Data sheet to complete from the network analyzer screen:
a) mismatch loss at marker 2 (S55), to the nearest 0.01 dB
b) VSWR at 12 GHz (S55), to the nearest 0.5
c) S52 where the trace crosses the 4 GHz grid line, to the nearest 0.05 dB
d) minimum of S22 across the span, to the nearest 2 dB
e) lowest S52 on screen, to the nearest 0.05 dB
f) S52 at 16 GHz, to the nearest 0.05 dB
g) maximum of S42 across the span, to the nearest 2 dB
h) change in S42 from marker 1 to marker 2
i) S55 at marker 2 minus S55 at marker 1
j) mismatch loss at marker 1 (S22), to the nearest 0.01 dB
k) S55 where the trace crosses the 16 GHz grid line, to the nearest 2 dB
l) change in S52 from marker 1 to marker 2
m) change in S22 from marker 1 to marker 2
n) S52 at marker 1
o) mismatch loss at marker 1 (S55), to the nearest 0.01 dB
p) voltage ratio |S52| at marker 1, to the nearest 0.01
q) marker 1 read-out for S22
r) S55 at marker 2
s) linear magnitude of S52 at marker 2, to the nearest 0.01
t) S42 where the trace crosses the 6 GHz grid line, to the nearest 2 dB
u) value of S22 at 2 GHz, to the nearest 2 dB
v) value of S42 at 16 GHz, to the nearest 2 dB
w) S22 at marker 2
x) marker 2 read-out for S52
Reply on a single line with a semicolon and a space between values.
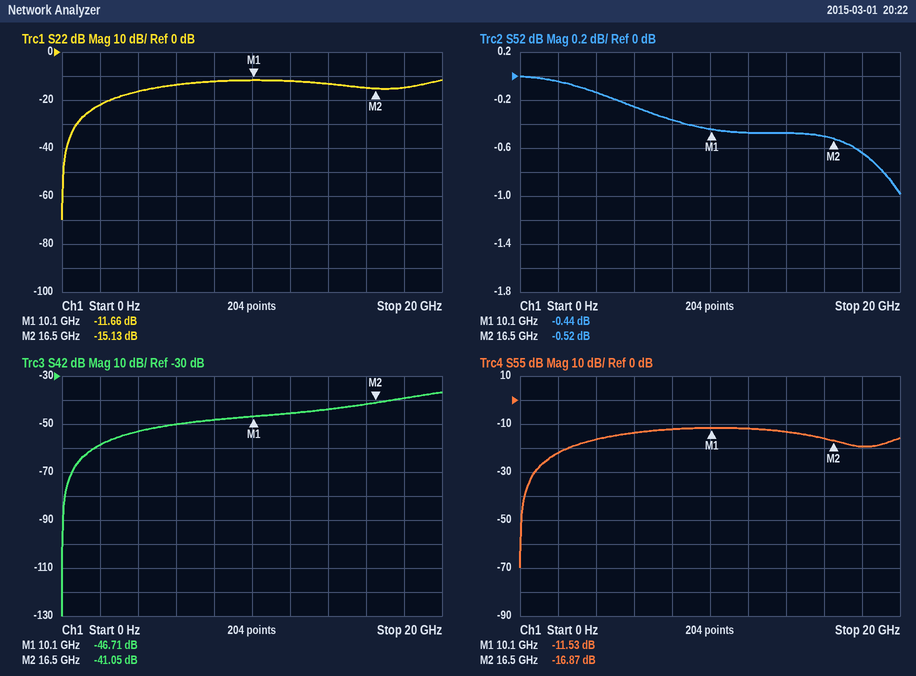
0.09 dB; 1.5; -0.15 dB; -70 dB; -1.00 dB; -0.50 dB; -36 dB; 5.66 dB; -5.34 dB; 0.31 dB; -16 dB; -0.08 dB; -3.47 dB; -0.44 dB; 0.32 dB; 0.95; -11.66 dB; -16.87 dB; 0.94; -50 dB; -22 dB; -42 dB; -15.13 dB; -0.52 dB
